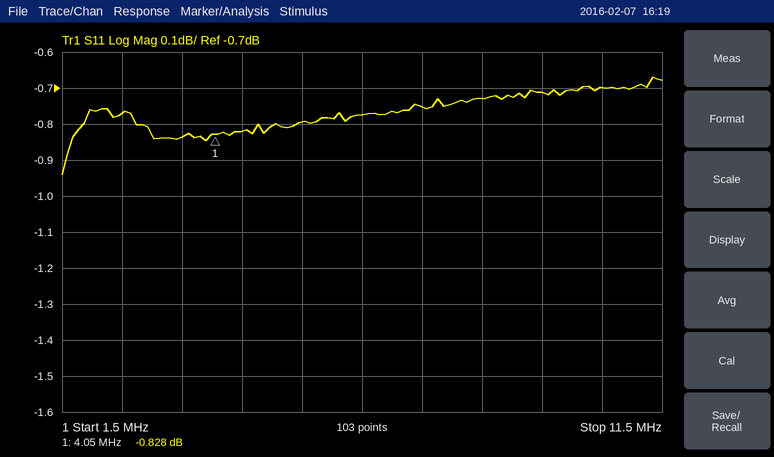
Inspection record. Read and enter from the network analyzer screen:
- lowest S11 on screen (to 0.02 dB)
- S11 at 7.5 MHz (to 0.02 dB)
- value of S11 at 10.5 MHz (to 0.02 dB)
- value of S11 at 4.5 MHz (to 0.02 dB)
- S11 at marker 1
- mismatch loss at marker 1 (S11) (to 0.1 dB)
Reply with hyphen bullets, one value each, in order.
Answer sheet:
- -0.94 dB
- -0.76 dB
- -0.70 dB
- -0.82 dB
- -0.828 dB
- 7.6 dB
